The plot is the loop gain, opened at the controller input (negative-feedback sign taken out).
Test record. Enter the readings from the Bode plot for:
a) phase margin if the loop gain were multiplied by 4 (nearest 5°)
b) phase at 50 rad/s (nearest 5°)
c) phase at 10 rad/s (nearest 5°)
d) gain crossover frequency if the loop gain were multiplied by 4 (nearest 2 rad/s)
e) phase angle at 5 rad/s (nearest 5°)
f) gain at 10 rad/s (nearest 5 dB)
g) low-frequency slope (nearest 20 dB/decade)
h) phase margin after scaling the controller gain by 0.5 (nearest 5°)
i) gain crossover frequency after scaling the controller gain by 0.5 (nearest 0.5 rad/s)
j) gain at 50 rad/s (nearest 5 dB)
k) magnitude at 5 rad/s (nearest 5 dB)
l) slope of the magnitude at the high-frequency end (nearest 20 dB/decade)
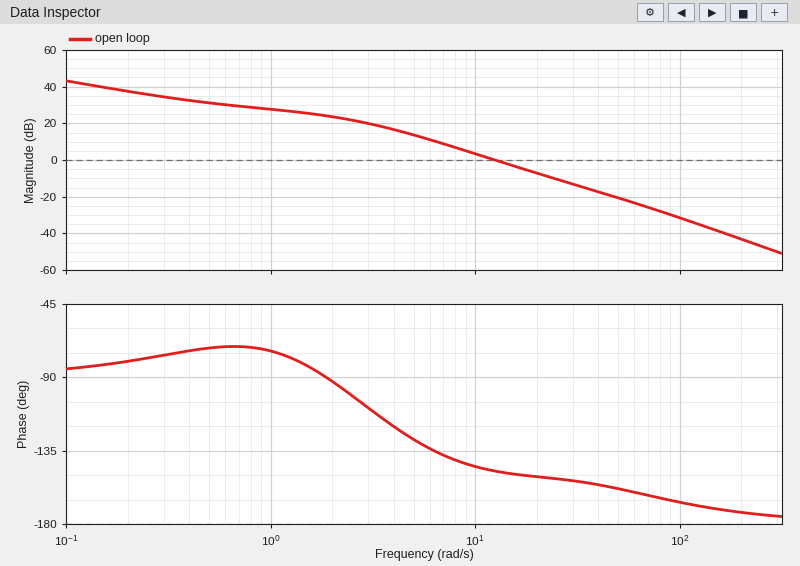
25°
-160°
-145°
28 rad/s
-130°
5 dB
-20 dB/decade
40°
8.5 rad/s
-20 dB
15 dB
-40 dB/decade
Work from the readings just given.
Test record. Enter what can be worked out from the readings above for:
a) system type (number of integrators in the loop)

1
